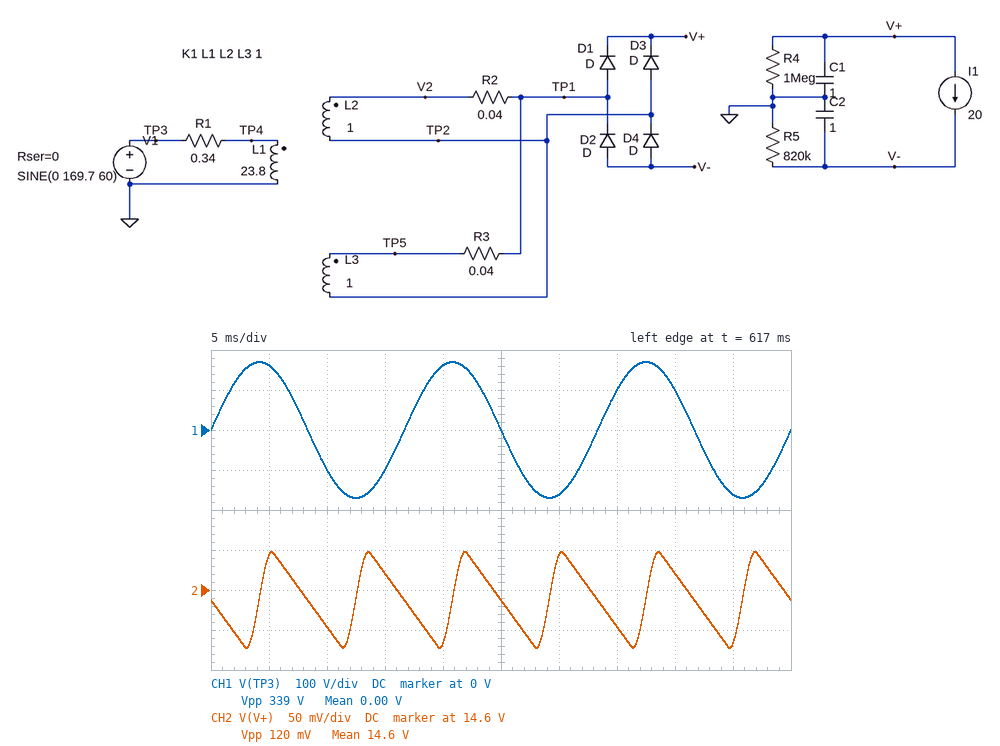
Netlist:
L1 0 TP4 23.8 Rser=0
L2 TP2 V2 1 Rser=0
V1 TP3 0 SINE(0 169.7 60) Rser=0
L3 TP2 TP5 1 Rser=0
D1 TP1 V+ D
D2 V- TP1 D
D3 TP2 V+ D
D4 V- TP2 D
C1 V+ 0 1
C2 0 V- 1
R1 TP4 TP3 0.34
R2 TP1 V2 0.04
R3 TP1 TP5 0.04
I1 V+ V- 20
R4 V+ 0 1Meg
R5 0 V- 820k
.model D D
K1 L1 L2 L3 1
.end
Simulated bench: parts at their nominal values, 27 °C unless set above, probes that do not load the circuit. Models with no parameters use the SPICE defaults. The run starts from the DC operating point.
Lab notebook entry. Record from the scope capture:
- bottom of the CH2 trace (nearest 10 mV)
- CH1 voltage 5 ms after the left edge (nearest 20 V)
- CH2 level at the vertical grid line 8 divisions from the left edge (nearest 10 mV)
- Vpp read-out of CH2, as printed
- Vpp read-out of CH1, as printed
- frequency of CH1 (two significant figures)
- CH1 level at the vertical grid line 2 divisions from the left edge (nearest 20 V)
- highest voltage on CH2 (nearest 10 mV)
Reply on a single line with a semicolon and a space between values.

14.53 V; 160 V; 14.62 V; 120 mV; 339 V; 60 Hz; -100 V; 14.65 V
